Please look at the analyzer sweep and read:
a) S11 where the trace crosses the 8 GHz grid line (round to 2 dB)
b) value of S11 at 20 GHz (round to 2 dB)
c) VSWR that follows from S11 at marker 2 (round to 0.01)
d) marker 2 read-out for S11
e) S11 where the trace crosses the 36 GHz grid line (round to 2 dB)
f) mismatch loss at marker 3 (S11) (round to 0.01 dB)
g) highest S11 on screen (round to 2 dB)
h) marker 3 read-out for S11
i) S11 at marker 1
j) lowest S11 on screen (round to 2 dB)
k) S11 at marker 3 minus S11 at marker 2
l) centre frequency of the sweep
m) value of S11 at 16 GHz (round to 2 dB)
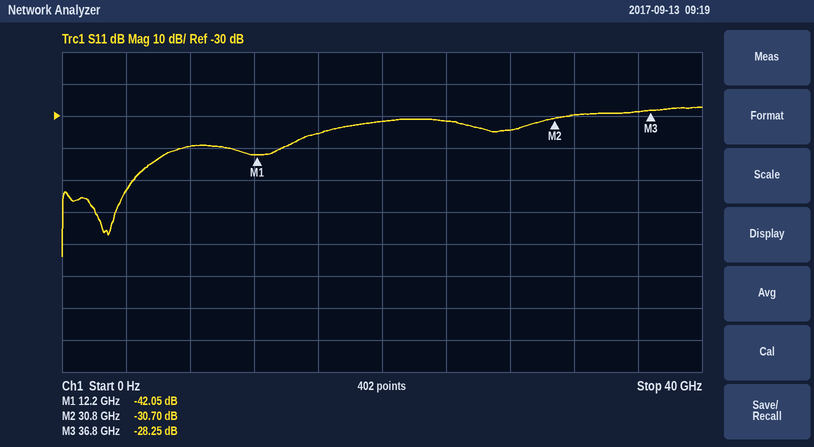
-40 dB
-32 dB
1.06
-30.70 dB
-28 dB
0.01 dB
-28 dB
-28.25 dB
-42.05 dB
-74 dB
2.45 dB
20 GHz
-36 dB
